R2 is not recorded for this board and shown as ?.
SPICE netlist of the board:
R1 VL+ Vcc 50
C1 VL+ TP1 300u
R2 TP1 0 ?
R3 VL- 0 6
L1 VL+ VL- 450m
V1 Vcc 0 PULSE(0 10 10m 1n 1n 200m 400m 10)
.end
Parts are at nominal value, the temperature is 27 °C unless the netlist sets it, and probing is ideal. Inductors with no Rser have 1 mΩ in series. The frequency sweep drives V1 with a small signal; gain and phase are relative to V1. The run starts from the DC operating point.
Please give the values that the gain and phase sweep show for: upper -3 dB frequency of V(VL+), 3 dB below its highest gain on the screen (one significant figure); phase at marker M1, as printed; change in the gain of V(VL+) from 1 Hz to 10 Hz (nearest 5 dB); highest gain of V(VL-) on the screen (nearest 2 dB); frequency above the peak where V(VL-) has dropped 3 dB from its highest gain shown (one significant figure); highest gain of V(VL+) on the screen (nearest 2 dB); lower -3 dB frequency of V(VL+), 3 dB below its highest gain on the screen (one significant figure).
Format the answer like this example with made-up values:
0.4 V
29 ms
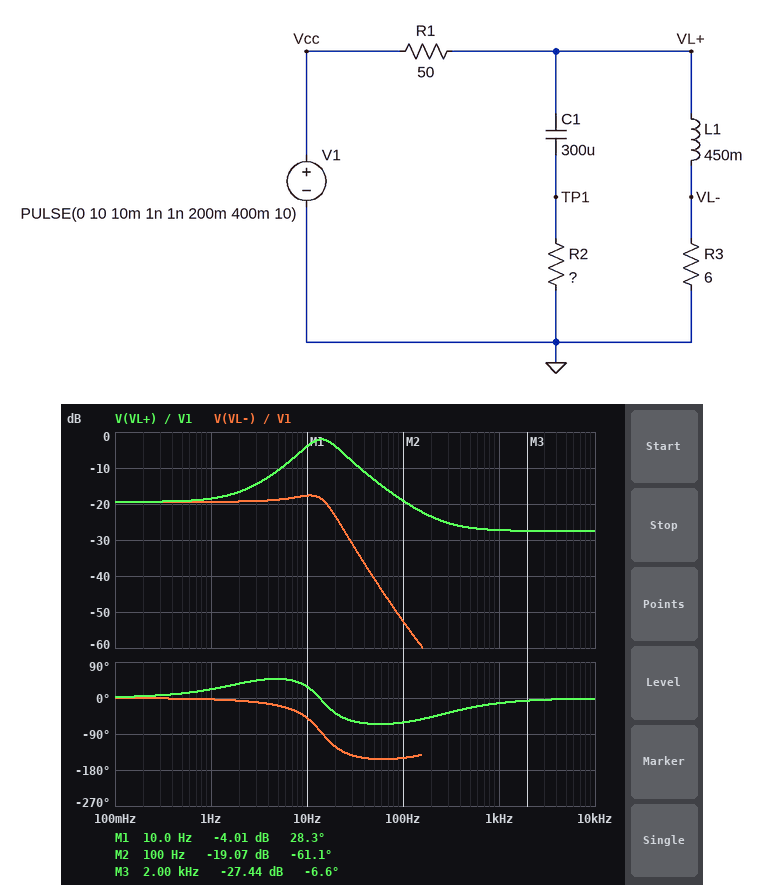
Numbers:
20 Hz
28.3 deg
15 dB
-18 dB
20 Hz
-2 dB
9 Hz
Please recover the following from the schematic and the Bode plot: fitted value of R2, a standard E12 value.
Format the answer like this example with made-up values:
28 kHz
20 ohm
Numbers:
2.2 Ω
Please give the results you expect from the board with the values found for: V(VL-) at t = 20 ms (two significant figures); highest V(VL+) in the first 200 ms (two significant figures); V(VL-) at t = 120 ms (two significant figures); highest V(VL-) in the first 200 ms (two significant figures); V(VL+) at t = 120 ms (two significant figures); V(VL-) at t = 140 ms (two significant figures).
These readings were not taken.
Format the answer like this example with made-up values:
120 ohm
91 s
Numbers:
340 mV
4.6 V
1.1 V
1.3 V
1.1 V
1.1 V
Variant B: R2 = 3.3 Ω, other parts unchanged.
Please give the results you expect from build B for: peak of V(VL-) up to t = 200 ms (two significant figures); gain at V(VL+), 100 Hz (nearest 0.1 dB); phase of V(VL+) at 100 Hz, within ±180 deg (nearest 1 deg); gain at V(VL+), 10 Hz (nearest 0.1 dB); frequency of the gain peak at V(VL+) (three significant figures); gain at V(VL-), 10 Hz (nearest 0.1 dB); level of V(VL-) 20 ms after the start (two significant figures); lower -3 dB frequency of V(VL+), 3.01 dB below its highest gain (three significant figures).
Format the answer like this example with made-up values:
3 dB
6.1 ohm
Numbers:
1.3 V
-18.5 dB
-52 deg
-4.1 dB
14.0 Hz
-17.8 dB
350 mV
8.81 Hz
